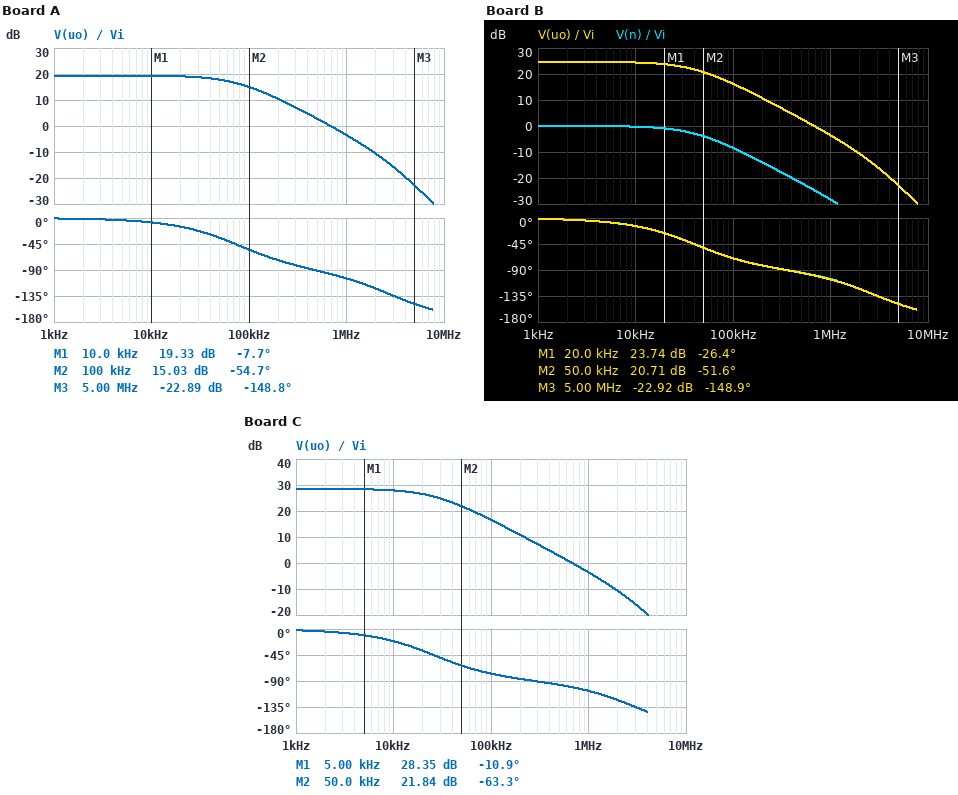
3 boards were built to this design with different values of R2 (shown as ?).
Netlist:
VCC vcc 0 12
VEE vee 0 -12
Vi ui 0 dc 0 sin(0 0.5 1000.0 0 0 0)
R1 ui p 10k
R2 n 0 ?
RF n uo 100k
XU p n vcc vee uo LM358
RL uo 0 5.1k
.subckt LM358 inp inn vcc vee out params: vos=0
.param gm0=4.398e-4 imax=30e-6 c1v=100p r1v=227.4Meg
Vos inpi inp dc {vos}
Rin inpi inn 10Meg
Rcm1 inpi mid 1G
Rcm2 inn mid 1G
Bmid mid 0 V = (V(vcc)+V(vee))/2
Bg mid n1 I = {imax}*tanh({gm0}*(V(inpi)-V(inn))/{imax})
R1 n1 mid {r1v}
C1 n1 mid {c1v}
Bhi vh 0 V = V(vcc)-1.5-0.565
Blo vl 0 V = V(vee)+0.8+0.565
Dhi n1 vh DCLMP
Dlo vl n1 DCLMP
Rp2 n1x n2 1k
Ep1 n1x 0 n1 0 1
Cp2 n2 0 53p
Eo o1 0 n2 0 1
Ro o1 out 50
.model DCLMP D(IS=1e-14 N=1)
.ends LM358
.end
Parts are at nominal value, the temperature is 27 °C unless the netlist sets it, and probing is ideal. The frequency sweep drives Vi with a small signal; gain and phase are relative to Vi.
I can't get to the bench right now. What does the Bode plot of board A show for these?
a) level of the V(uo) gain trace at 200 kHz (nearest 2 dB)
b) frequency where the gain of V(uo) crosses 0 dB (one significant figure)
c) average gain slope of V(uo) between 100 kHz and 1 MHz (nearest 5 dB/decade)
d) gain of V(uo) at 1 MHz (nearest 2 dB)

10 dB
700 kHz
-20 dB/decade
-4 dB
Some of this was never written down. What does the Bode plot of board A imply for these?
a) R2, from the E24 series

12 kΩ
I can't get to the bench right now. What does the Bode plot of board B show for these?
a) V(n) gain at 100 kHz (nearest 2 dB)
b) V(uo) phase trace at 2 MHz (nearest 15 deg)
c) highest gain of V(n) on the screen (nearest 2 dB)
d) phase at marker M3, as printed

-8 dB
-120 deg
0 dB
-148.9 deg
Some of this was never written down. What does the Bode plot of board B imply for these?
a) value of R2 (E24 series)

6.2 kΩ
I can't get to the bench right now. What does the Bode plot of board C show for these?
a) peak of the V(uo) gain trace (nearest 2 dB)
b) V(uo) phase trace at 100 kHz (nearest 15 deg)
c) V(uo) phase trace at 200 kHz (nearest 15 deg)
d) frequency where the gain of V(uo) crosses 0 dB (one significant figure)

28 dB
-75 deg
-90 deg
700 kHz
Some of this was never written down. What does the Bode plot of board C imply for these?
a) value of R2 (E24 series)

3.9 kΩ
